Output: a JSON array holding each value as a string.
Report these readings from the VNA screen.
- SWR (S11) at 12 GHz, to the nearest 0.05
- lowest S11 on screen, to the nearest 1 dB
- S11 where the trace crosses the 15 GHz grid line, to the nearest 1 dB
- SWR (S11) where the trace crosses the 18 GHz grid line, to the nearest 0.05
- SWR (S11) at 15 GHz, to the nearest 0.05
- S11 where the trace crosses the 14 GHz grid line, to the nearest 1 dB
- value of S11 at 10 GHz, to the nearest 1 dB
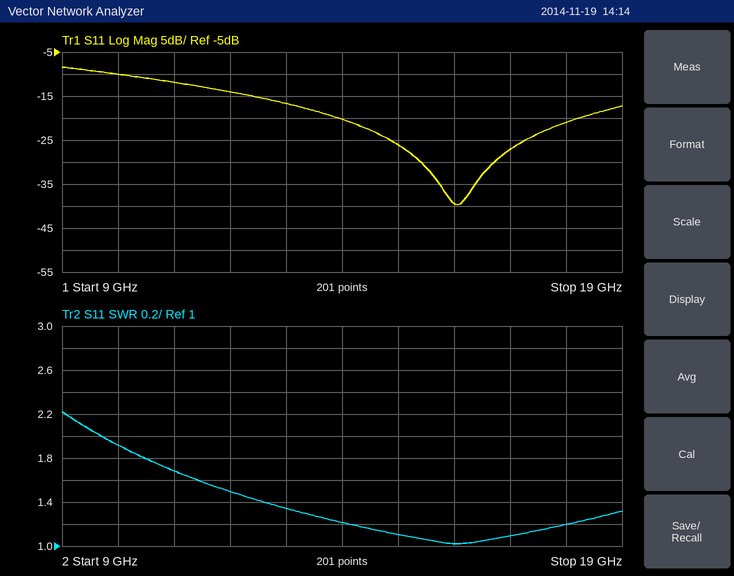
["1.50", "-40 dB", "-26 dB", "1.20", "1.10", "-20 dB", "-10 dB"]
